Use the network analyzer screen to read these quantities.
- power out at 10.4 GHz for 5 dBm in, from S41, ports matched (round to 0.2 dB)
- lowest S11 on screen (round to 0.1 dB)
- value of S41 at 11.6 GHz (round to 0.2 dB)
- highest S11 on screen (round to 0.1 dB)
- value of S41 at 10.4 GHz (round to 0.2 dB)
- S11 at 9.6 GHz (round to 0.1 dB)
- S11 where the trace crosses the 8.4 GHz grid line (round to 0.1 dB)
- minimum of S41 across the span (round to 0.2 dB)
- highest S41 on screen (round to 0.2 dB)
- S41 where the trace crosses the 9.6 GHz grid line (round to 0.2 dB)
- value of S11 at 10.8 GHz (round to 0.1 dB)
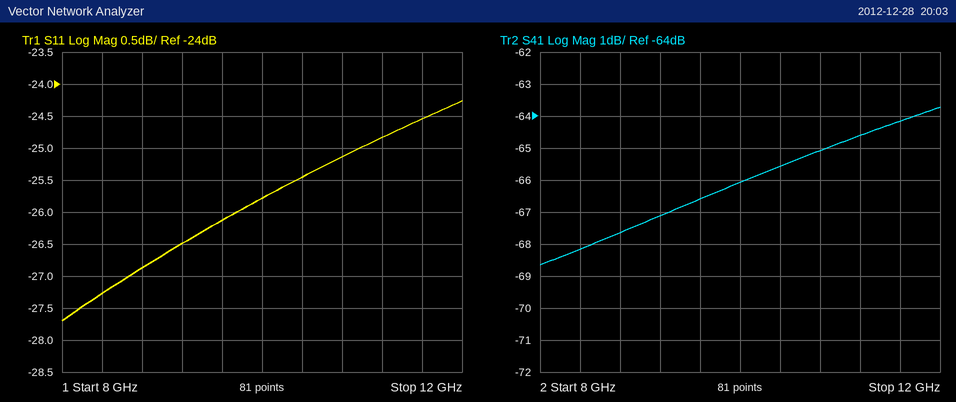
-60.6 dBm
-27.7 dB
-64.2 dB
-24.3 dB
-65.6 dB
-26.1 dB
-27.3 dB
-68.6 dB
-63.8 dB
-66.6 dB
-25.1 dB
